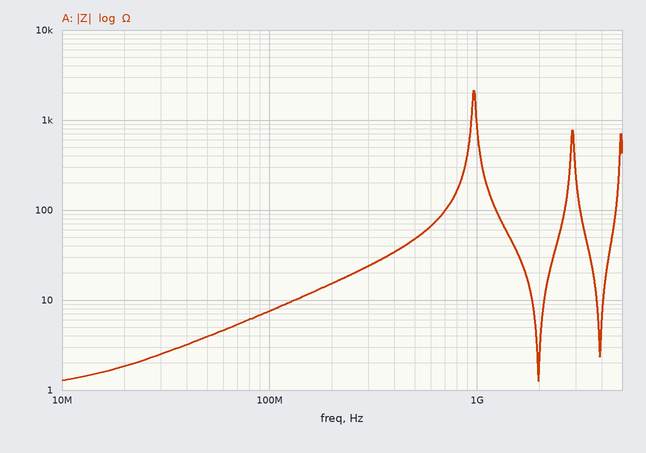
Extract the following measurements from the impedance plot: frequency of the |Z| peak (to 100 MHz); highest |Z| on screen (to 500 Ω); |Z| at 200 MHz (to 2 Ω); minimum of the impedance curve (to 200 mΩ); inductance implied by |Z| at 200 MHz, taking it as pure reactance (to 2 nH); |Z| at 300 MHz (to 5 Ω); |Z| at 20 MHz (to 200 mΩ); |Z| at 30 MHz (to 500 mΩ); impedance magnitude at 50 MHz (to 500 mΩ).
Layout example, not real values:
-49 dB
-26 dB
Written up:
1.0 GHz
2.0 kΩ
16 Ω
1.2 Ω
12 nH
25 Ω
1.8 Ω
2.5 Ω
4.0 Ω
